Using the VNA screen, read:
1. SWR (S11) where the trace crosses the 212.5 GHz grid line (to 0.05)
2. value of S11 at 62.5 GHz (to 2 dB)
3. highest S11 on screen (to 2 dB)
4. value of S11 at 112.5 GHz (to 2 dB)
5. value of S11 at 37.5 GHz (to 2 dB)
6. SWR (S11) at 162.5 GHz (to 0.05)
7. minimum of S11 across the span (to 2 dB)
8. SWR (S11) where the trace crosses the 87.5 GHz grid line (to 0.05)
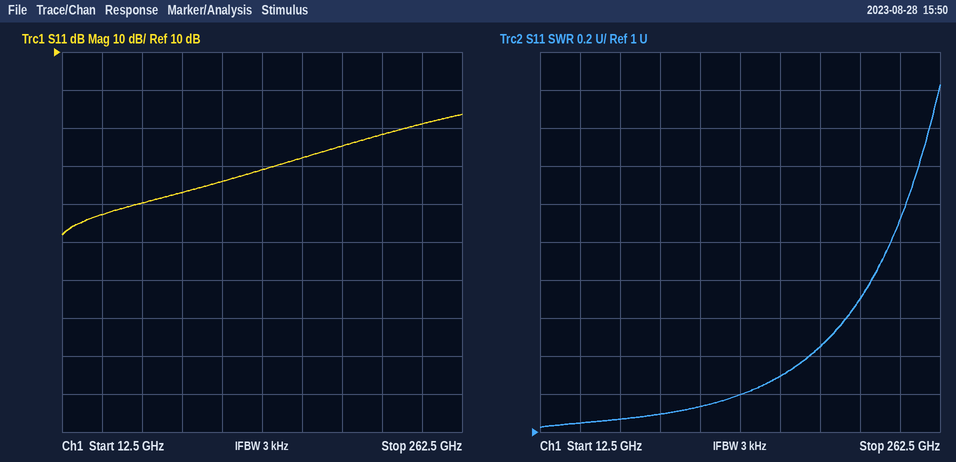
1.70
-30 dB
-6 dB
-24 dB
-32 dB
1.30
-38 dB
1.10
